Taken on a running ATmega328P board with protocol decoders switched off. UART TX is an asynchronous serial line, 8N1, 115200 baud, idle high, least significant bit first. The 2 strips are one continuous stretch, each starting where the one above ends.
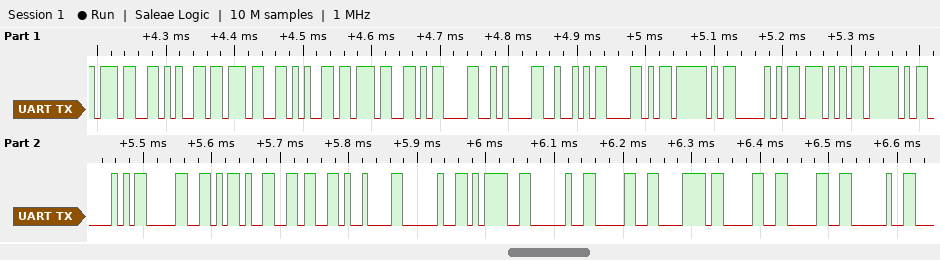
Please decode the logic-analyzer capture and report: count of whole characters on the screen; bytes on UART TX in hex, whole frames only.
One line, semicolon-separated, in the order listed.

26; 37 65 37 65 37 0D 0A 52 58 5F 50 57 5F 50 30 2D 36 09 20 3D 20 30 78 30 30 20
